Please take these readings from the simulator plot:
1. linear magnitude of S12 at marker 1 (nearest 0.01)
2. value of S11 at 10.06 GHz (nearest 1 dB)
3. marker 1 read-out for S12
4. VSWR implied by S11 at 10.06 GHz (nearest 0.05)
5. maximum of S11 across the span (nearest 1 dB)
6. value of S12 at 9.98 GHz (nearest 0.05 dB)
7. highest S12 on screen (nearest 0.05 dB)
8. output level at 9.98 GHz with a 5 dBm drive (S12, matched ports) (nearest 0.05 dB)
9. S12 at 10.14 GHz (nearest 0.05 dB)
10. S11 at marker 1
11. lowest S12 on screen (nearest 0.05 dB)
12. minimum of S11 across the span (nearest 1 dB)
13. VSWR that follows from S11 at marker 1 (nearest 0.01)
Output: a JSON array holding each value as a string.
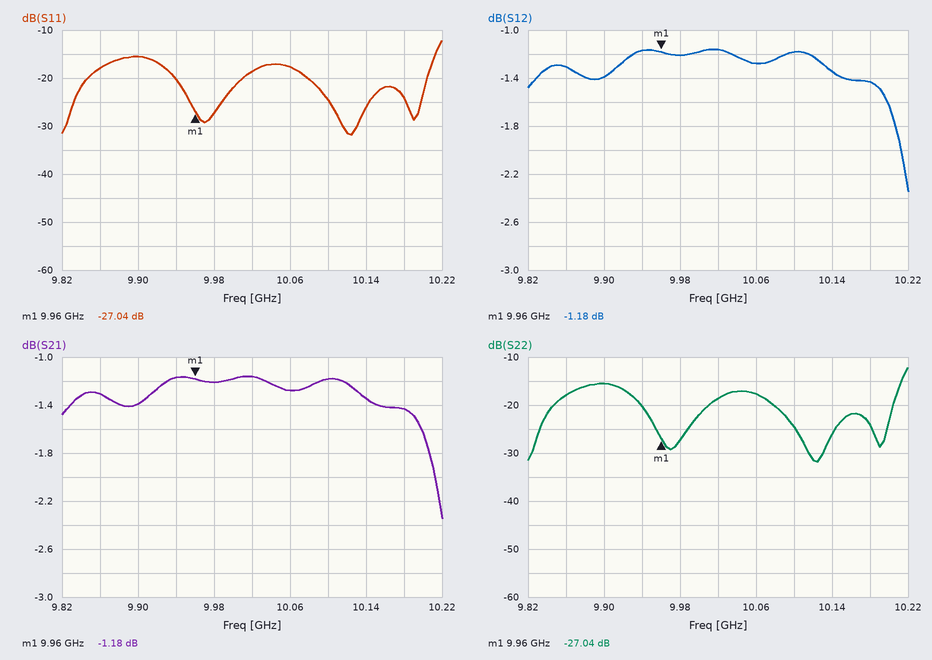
["0.87", "-18 dB", "-1.18 dB", "1.30", "-12 dB", "-1.20 dB", "-1.15 dB", "3.80 dBm", "-1.35 dB", "-27.04 dB", "-2.35 dB", "-32 dB", "1.09"]
